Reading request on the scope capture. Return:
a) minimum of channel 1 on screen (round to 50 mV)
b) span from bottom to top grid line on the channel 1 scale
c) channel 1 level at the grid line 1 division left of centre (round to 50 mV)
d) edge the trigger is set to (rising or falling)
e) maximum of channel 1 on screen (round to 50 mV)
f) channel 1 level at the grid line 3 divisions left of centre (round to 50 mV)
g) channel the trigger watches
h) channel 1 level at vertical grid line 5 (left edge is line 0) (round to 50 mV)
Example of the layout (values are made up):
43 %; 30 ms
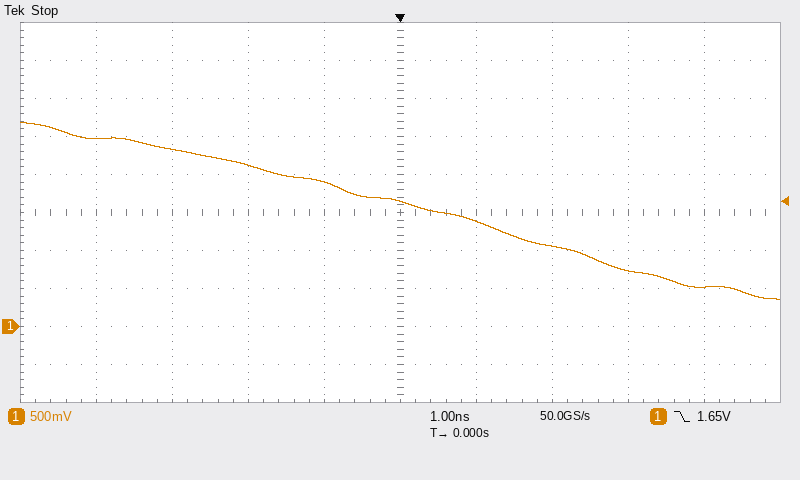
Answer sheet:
350 mV; 5 V; 1.90 V; falling; 2.70 V; 2.35 V; channel 1; 1.65 V
